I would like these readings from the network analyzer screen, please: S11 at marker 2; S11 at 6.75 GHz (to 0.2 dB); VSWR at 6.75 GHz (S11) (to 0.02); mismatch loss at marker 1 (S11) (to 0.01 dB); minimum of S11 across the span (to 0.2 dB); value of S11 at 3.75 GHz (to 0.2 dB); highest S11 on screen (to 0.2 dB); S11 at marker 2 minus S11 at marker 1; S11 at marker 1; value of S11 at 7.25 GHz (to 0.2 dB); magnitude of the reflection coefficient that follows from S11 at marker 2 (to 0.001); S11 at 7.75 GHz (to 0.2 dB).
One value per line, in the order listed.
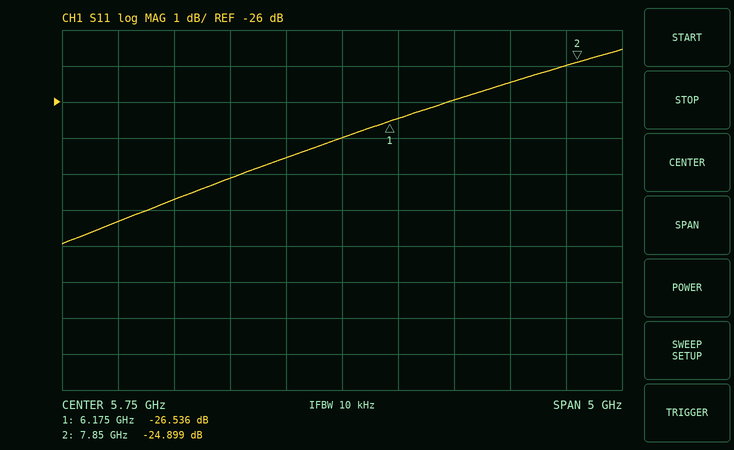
-24.899 dB
-26.0 dB
1.10
0.01 dB
-30.0 dB
-29.4 dB
-24.6 dB
1.637 dB
-26.536 dB
-25.4 dB
0.057
-25.0 dB
